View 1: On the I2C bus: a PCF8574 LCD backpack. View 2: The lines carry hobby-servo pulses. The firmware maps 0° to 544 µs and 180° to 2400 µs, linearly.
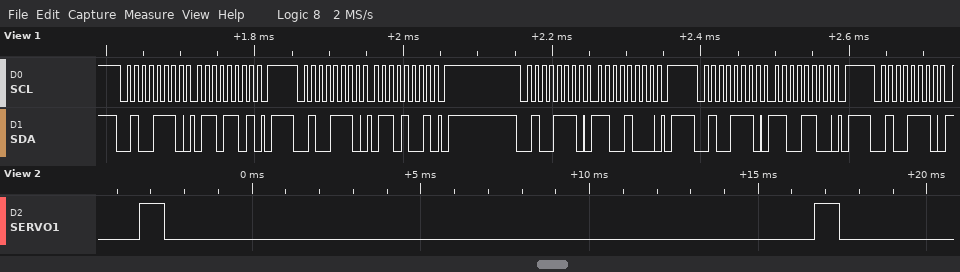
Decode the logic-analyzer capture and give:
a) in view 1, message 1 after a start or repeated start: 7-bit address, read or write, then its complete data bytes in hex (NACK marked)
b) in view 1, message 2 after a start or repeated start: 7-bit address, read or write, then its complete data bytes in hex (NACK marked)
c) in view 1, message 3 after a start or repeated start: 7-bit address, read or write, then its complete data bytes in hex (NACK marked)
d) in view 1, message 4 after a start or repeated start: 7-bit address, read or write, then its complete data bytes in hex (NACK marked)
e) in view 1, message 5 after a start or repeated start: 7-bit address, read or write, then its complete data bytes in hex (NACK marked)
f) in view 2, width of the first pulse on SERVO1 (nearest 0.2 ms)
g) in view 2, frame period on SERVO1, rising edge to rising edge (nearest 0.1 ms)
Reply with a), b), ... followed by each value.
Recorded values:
a) 0x27 write: 6D
b) 0x27 write: 69
c) 0x27 write: C8
d) 0x27 write: CC
e) 0x27 write
f) 0.8 ms
g) 20.0 ms
